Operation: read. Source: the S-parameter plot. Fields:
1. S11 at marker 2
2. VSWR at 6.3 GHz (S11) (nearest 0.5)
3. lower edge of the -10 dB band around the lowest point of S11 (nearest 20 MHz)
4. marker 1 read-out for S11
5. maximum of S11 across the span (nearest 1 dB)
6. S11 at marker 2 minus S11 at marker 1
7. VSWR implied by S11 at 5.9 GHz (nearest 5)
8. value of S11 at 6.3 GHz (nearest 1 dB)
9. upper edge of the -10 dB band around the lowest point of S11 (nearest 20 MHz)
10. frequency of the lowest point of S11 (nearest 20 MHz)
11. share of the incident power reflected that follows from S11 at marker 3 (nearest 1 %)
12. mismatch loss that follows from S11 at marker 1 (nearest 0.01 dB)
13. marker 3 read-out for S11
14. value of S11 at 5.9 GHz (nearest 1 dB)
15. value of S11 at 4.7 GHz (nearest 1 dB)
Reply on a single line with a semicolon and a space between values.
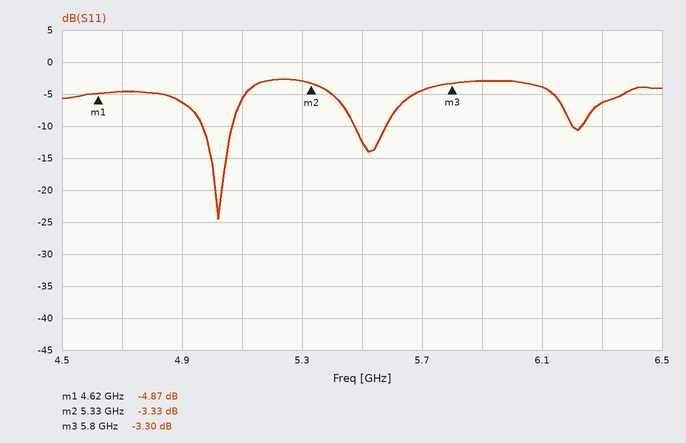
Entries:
-3.33 dB; 3.0; 4.96 GHz; -4.87 dB; -3 dB; 1.54 dB; 5; -6 dB; 5.06 GHz; 5.02 GHz; 47 %; 1.71 dB; -3.30 dB; -3 dB; -5 dB
